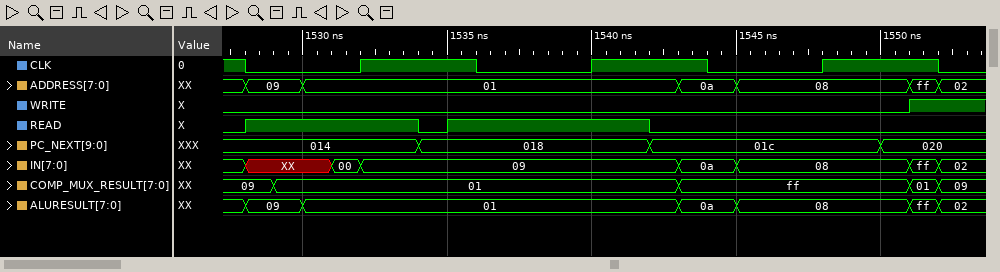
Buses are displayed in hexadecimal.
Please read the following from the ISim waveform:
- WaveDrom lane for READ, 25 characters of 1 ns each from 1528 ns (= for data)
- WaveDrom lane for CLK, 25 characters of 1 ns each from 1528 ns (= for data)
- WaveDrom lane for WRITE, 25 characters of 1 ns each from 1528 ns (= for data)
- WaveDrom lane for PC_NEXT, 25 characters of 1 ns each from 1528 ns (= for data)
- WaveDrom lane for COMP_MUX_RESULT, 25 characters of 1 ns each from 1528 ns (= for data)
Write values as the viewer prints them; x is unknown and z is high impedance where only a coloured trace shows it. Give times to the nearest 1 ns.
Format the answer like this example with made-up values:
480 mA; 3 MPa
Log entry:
{name: 'READ', wave: '1.....01......0..........'}; {name: 'CLK', wave: '0...1...0...1...0...1...0'}; {name: 'WRITE', wave: '0......................1.'}; {name: 'PC_NEXT', wave: '=.....=.......=.......=..', data: '014 018 01c 020'}; {name: 'COMP_MUX_RESULT', wave: '==.............=.......==', data: '09 01 ff 01 09'}
